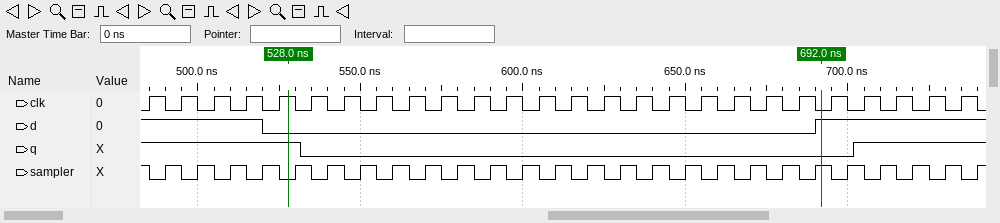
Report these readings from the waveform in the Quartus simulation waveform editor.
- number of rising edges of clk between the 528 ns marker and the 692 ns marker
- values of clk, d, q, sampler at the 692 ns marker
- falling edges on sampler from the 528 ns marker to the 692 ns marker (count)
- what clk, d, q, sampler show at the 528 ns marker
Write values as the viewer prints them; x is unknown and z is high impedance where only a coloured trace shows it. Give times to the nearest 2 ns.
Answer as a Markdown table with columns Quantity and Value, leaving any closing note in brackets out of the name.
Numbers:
| Quantity | Value |
|---|---|
| number of rising edges of clk between the 528 ns marker and the 692 ns marker | 16 |
| values of clk, d, q, sampler at the 692 ns marker | clk=0, d=1, q=0, sampler=1 |
| falling edges on sampler from the 528 ns marker to the 692 ns marker | 16 |
| what clk, d, q, sampler show at the 528 ns marker | clk=1, d=0, q=1, sampler=0 |
